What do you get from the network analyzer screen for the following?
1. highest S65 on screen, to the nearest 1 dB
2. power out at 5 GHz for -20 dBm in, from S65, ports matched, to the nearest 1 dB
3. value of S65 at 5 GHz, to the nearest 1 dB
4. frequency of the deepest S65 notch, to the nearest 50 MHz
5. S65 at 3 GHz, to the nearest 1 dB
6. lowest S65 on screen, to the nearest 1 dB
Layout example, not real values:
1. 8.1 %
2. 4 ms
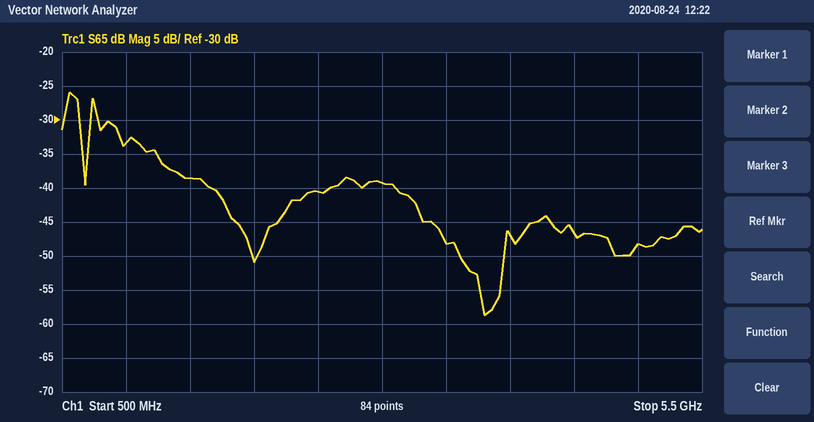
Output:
1. -26 dB
2. -68 dBm
3. -48 dB
4. 3.80 GHz
5. -39 dB
6. -59 dB
